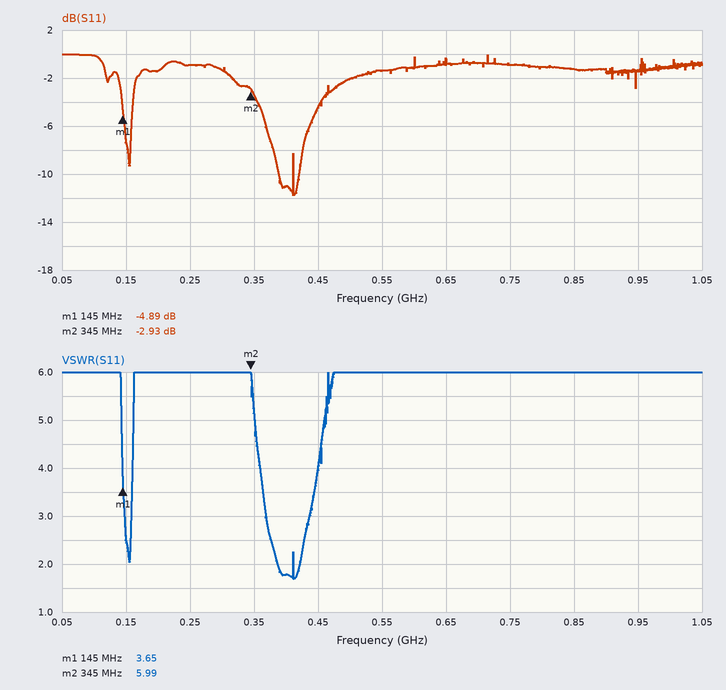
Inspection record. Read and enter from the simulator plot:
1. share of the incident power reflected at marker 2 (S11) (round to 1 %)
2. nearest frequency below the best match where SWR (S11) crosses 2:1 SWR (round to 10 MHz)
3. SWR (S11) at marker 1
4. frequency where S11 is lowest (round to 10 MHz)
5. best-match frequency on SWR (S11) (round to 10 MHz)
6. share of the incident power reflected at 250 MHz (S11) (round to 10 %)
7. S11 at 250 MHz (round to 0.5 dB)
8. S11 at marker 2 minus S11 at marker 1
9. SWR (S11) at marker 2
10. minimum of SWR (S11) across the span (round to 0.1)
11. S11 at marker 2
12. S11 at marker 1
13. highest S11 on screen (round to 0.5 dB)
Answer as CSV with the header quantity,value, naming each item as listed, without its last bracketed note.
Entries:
quantity,value
share of the incident power reflected at marker 2 (S11),51 %
nearest frequency below the best match where SWR (S11) crosses 2:1 SWR,390 MHz
SWR (S11) at marker 1,3.65
frequency where S11 is lowest,410 MHz
best-match frequency on SWR (S11),410 MHz
share of the incident power reflected at 250 MHz (S11),80 %
S11 at 250 MHz,-1.0 dB
S11 at marker 2 minus S11 at marker 1,1.96 dB
SWR (S11) at marker 2,5.99
minimum of SWR (S11) across the span,1.7
S11 at marker 2,-2.93 dB
S11 at marker 1,-4.89 dB
highest S11 on screen,0.0 dB
